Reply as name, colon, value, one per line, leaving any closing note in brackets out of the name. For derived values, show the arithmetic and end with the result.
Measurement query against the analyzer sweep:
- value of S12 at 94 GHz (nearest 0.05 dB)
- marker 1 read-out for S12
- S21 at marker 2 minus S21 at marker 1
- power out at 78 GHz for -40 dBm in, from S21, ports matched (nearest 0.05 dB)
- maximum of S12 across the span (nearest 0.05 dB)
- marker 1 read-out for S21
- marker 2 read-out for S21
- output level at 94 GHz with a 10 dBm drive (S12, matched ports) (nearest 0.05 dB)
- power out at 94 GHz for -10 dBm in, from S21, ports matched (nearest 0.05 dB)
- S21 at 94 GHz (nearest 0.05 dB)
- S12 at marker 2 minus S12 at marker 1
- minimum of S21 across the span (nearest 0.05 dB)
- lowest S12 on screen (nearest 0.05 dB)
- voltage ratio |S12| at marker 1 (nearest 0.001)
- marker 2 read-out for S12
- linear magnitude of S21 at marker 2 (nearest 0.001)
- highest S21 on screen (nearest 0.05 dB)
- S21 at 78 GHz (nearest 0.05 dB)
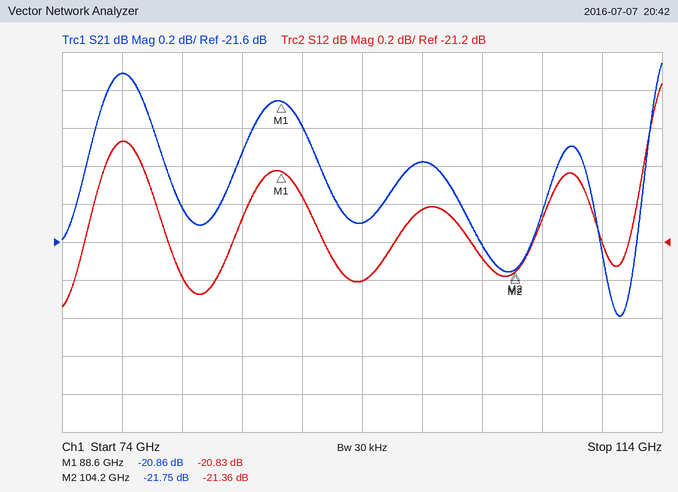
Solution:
value of S12 at 94 GHz: -21.40 dB
marker 1 read-out for S12: -20.83 dB
S21 at marker 2 minus S21 at marker 1: -21.75 − (-20.86) = -0.89 dB
power out at 78 GHz for -40 dBm in, from S21, ports matched: -40 dBm + (-20.70 dB) = -60.70 dBm
maximum of S12 across the span: -20.35 dB
marker 1 read-out for S21: -20.86 dB
marker 2 read-out for S21: -21.75 dB
output level at 94 GHz with a 10 dBm drive (S12, matched ports): 10 dBm + (-21.40 dB) = -11.40 dBm
power out at 94 GHz for -10 dBm in, from S21, ports matched: -10 dBm + (-21.50 dB) = -31.50 dBm
S21 at 94 GHz: -21.50 dB
S12 at marker 2 minus S12 at marker 1: -21.36 − (-20.83) = -0.53 dB
minimum of S21 across the span: -22.00 dB
lowest S12 on screen: -21.55 dB
voltage ratio |S12| at marker 1: 10^(-20.83/20) ≈ 0.091
marker 2 read-out for S12: -21.36 dB
linear magnitude of S21 at marker 2: 10^(-21.75/20) ≈ 0.082
highest S21 on screen: -20.65 dB
S21 at 78 GHz: -20.70 dB
